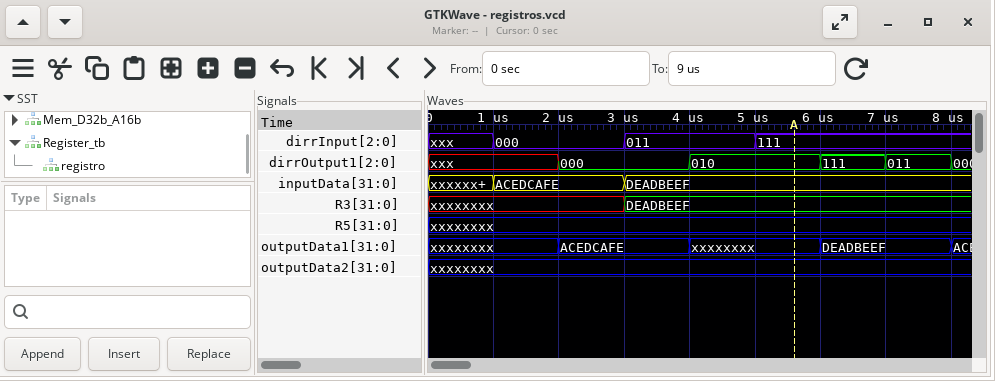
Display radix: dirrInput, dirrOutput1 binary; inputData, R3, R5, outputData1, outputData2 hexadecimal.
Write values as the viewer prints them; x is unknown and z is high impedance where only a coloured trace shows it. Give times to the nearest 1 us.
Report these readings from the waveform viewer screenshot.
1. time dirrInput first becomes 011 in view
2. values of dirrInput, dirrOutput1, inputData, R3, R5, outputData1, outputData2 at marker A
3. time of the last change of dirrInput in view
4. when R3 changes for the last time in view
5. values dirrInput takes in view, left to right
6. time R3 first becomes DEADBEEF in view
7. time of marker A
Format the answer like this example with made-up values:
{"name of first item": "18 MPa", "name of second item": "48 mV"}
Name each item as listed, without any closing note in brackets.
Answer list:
{"time dirrInput first becomes 011 in view": "3 us", "values of dirrInput, dirrOutput1, inputData, R3, R5, outputData1, outputData2 at marker A": "dirrInput=111, dirrOutput1=010, inputData=DEADBEEF, R3=DEADBEEF, R5=xxxxxxxx, outputData1=xxxxxxxx, outputData2=xxxxxxxx", "time of the last change of dirrInput in view": "5 us", "when R3 changes for the last time in view": "3 us", "values dirrInput takes in view, left to right": "xxx, 000, 011, 111", "time R3 first becomes DEADBEEF in view": "3 us", "time of marker A": "6 us"}
